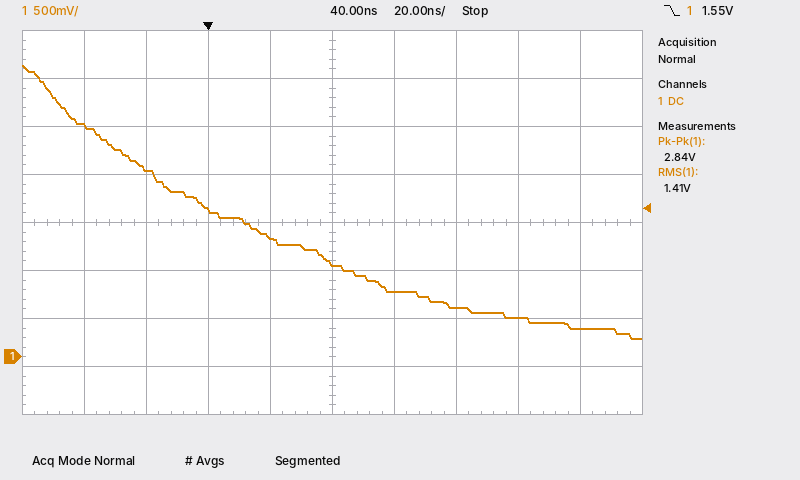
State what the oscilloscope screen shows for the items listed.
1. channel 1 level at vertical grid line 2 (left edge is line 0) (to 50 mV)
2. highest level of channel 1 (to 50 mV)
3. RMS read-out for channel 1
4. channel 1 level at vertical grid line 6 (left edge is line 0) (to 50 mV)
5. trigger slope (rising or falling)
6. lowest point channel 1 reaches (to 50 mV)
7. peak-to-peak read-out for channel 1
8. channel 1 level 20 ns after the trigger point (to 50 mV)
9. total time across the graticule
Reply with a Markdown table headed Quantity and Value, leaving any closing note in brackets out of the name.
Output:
| Quantity | Value |
|---|---|
| channel 1 level at vertical grid line 2 (left edge is line 0) | 1.95 V |
| highest level of channel 1 | 3.05 V |
| RMS read-out for channel 1 | 1.41 V |
| channel 1 level at vertical grid line 6 (left edge is line 0) | 700 mV |
| trigger slope | falling |
| lowest point channel 1 reaches | 200 mV |
| peak-to-peak read-out for channel 1 | 2.84 V |
| channel 1 level 20 ns after the trigger point | 1.25 V |
| total time across the graticule | 200 ns |
